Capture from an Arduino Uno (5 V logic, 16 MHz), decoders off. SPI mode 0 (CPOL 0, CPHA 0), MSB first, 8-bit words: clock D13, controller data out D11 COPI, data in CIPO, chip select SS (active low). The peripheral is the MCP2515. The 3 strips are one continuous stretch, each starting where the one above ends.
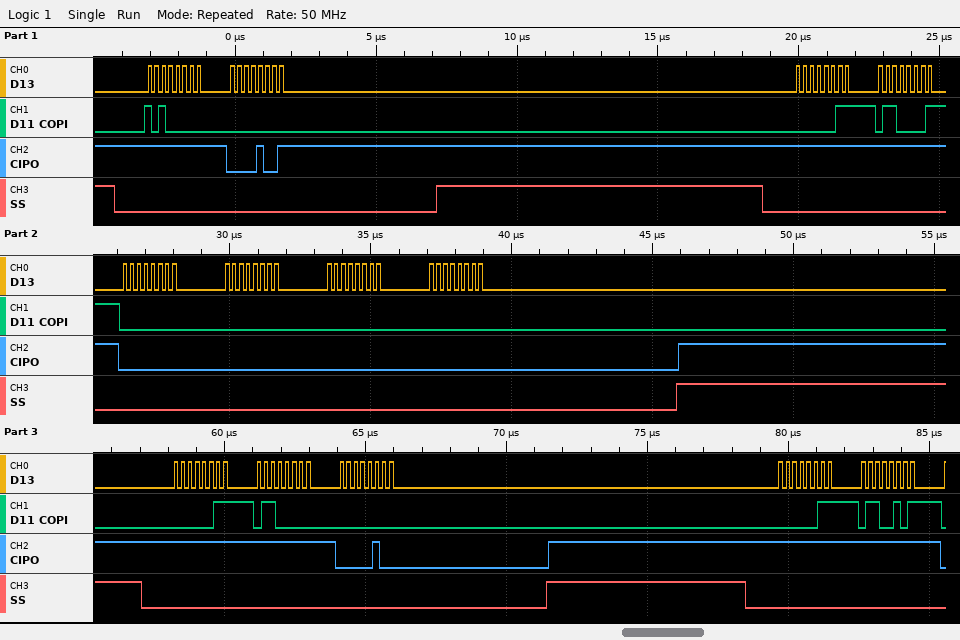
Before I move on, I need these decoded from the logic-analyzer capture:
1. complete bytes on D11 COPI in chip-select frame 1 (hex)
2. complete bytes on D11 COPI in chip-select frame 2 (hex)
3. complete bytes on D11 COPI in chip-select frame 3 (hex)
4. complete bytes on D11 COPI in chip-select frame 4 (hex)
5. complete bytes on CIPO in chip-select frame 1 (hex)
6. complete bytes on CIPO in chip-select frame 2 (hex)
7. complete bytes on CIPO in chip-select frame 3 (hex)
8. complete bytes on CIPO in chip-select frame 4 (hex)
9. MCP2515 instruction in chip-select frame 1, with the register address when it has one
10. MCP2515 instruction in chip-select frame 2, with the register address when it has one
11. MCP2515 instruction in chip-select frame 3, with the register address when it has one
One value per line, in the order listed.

A0 00
03 61 00 00 00 00
03 60 00
03 65
FF 09
FF FF 00 00 00 00
FF FF 04
FF FF
READ STATUS
READ 0x61
READ 0x60
